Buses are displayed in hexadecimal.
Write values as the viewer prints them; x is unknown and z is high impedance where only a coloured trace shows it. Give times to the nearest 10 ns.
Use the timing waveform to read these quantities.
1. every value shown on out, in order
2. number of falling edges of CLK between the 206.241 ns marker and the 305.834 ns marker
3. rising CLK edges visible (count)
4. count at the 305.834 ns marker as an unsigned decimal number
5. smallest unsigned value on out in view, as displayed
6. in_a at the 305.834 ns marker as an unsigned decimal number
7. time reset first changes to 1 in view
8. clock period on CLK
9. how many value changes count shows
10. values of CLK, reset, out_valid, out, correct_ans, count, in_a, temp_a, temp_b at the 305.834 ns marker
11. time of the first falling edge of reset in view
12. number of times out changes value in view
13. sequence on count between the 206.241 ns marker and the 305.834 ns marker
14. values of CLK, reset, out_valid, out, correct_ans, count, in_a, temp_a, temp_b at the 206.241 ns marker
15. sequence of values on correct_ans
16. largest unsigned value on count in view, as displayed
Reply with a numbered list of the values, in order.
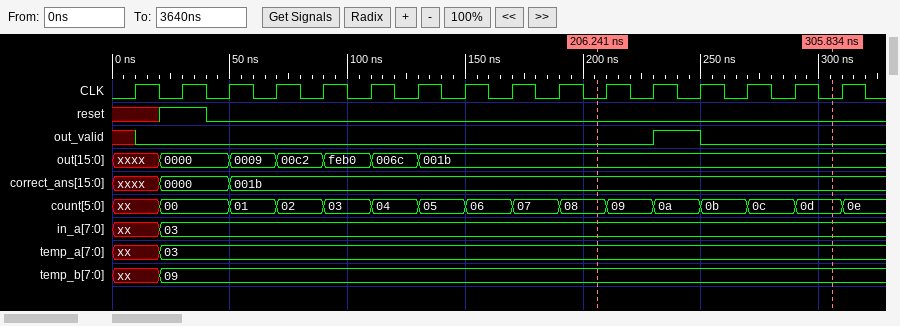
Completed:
1. xxxx, 0000, 0009, 00c2, feb0, 006c, 001b
2. 5
3. 16
4. 13
5. 0000
6. 3
7. 20 ns
8. 20 ns
9. 15
10. CLK=0, reset=0, out_valid=0, out=001b, correct_ans=001b, count=0d, in_a=03, temp_a=03, temp_b=09
11. 40 ns
12. 6
13. 08, 09, 0a, 0b, 0c, 0d
14. CLK=0, reset=0, out_valid=0, out=001b, correct_ans=001b, count=08, in_a=03, temp_a=03, temp_b=09
15. xxxx, 0000, 001b
16. 0e
